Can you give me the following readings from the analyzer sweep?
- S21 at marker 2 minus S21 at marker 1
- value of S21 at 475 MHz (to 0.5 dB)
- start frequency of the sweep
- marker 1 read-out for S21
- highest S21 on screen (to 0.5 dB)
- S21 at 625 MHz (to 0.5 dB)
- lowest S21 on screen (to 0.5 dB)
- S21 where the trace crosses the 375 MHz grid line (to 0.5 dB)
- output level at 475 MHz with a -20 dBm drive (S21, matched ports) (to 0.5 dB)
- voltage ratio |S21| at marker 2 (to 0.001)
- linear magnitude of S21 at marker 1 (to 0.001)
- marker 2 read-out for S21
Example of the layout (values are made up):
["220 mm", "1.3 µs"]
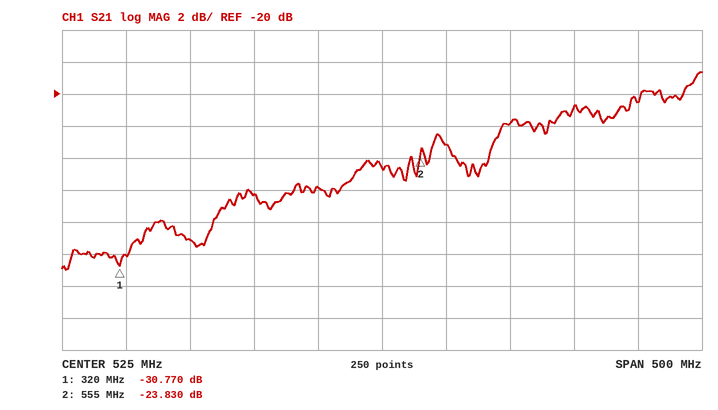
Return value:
["6.940 dB", "-26.0 dB", "275 MHz", "-30.770 dB", "-18.5 dB", "-22.0 dB", "-31.0 dB", "-29.0 dB", "-46.0 dBm", "0.064", "0.029", "-23.830 dB"]
